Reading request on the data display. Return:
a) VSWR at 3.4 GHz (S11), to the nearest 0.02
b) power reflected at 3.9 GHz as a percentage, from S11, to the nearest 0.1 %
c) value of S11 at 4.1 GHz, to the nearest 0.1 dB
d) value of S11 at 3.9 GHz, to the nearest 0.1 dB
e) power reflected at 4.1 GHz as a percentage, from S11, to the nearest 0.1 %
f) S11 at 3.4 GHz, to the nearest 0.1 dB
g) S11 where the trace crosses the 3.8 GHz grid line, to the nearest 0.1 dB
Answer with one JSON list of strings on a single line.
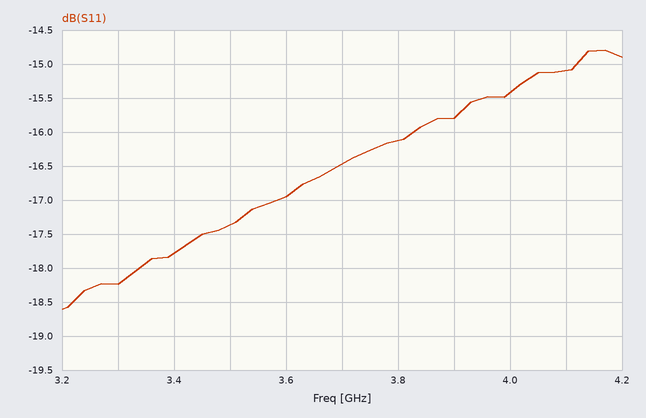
["1.30", "2.6 %", "-15.1 dB", "-15.8 dB", "3.1 %", "-17.8 dB", "-16.1 dB"]
